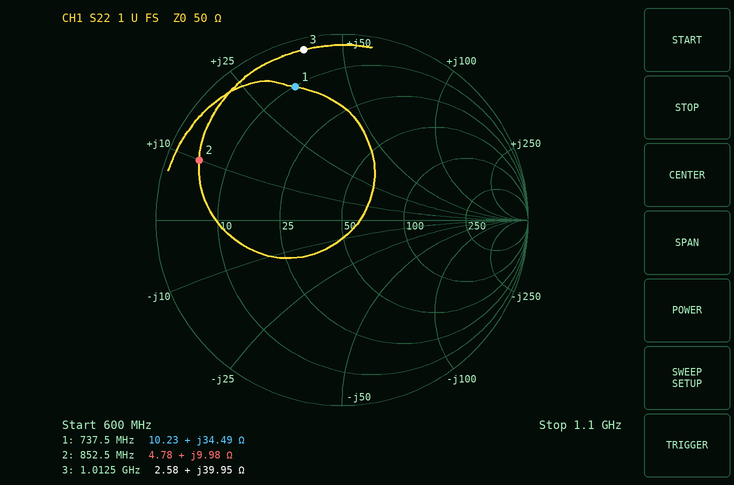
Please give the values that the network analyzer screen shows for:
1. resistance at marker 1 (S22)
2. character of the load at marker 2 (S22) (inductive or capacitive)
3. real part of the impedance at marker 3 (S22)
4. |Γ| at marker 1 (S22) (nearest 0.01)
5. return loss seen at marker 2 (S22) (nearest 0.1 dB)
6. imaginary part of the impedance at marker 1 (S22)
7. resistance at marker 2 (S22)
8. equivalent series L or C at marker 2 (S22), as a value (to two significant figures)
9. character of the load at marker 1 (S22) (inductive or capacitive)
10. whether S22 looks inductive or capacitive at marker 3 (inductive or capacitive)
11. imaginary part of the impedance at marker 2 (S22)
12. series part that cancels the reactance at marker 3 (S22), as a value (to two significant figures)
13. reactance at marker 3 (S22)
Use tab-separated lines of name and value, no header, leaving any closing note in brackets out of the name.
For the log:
resistance at marker 1	10.23 Ω
character of the load at marker 2 (S22)	inductive
real part of the impedance at marker 3	2.58 Ω
|Γ| at marker 1 (S22)	0.76
return loss seen at marker 2 (S22)	1.6 dB
imaginary part of the impedance at marker 1	+34.49 Ω
resistance at marker 2	4.78 Ω
equivalent series L or C at marker 2 (S22), as a value	1.9 nH
character of the load at marker 1 (S22)	inductive
whether S22 looks inductive or capacitive at marker 3	inductive
imaginary part of the impedance at marker 2	+9.98 Ω
series part that cancels the reactance at marker 3 (S22), as a value	3.9 pF
reactance at marker 3	+39.95 Ω
